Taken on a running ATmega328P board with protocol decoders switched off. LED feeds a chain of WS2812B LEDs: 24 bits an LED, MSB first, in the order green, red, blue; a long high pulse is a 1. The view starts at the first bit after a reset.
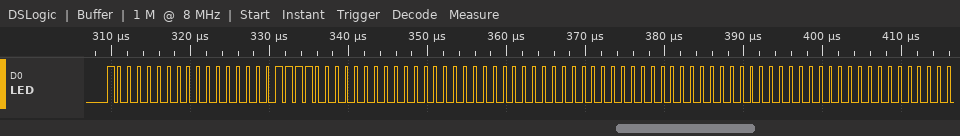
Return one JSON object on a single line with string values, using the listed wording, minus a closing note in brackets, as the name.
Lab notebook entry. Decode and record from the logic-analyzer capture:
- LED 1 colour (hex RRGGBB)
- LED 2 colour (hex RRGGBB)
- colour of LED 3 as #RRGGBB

{"LED 1 colour": "#008078", "LED 2 colour": "#000000", "colour of LED 3 as #RRGGBB": "#000000"}
